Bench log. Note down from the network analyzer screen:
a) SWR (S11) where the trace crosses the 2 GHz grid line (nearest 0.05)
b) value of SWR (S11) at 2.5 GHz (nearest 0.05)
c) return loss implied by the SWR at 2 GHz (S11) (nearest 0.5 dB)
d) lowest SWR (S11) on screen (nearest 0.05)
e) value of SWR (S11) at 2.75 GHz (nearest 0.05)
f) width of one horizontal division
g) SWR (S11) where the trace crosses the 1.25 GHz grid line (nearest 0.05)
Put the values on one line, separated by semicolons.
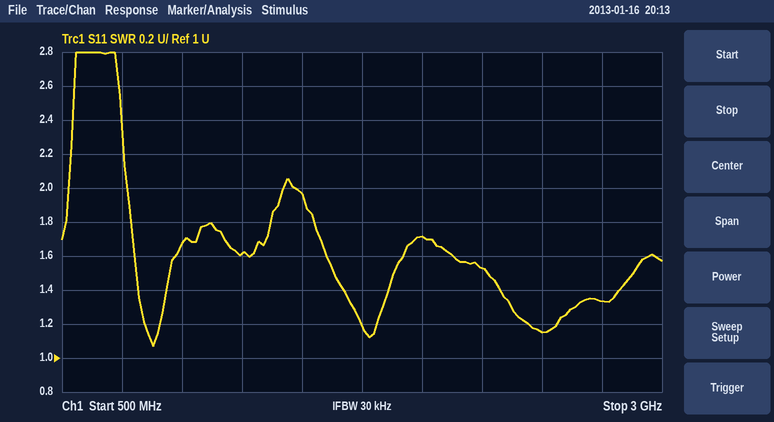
1.70; 1.15; 11.5 dB; 1.05; 1.35; 250 MHz; 1.60
